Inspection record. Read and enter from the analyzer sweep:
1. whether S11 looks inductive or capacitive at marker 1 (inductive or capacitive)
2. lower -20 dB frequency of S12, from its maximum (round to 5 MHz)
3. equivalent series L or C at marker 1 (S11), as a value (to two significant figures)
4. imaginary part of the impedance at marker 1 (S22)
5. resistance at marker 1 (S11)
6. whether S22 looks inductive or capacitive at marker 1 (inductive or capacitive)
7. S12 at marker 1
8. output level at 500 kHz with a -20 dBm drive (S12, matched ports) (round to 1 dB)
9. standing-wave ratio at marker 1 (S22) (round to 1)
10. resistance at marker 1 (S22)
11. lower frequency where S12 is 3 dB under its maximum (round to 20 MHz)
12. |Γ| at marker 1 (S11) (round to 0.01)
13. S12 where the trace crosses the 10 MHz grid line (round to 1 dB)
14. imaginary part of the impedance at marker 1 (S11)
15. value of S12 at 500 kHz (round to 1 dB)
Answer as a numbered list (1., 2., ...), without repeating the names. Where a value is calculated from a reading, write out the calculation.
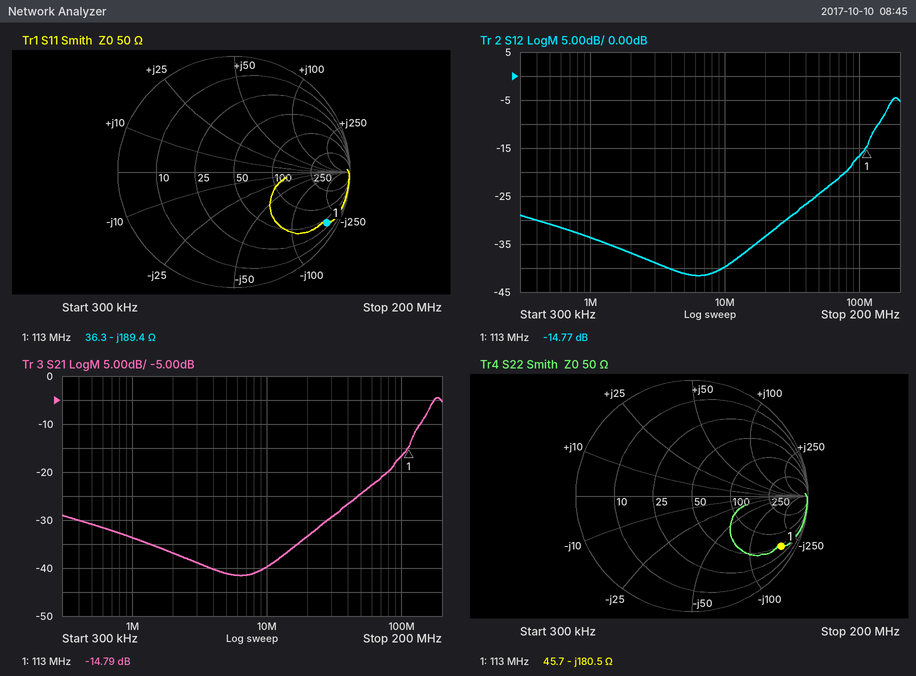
1. capacitive
2. 50 MHz
3. C = 1/(2π × 113 MHz × 189.4 Ω) ≈ 7.4 pF
4. -180.5 Ω
5. 36.3 Ω
6. capacitive
7. -14.77 dB
8. -20 dBm + (-31 dB) = -51 dBm
9. 16
10. 45.7 Ω
11. 160 MHz
12. 0.91
13. -40 dB
14. -189.4 Ω
15. -31 dB
